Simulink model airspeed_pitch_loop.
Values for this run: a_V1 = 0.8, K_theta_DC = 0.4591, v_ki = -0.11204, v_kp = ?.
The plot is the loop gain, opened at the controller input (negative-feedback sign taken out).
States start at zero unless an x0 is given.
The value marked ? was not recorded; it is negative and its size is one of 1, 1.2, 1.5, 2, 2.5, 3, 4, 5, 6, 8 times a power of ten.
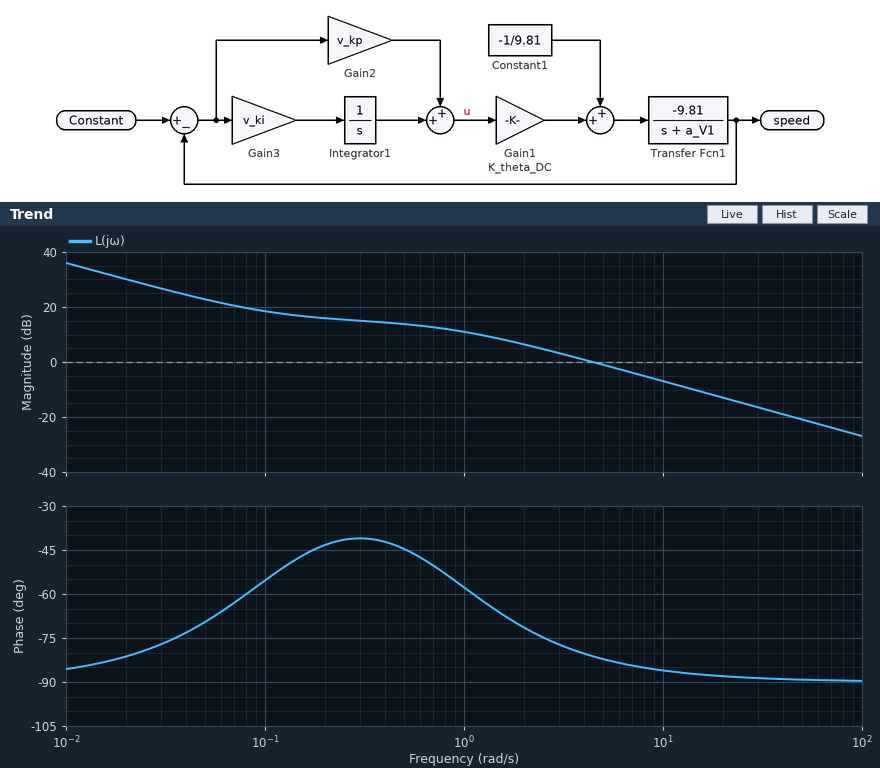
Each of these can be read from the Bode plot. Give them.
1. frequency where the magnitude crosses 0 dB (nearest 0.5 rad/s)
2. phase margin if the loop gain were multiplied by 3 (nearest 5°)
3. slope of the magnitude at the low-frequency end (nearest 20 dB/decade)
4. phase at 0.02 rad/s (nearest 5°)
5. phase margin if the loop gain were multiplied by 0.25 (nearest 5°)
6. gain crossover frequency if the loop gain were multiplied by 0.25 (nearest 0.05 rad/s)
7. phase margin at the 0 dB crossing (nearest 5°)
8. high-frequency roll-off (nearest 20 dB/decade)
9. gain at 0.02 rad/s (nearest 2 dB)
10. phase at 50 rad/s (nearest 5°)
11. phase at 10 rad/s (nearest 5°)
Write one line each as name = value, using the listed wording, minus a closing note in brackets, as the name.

frequency where the magnitude crosses 0 dB = 4.5 rad/s
phase margin if the loop gain were multiplied by 3 = 95°
slope of the magnitude at the low-frequency end = -20 dB/decade
phase at 0.02 rad/s = -80°
phase margin if the loop gain were multiplied by 0.25 = 125°
gain crossover frequency if the loop gain were multiplied by 0.25 = 0.80 rad/s
phase margin at the 0 dB crossing = 100°
high-frequency roll-off = -20 dB/decade
gain at 0.02 rad/s = 30 dB
phase at 50 rad/s = -90°
phase at 10 rad/s = -85°
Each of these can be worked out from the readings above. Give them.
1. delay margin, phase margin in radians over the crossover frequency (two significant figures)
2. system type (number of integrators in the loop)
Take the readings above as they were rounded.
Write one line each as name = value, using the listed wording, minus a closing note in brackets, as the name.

delay margin, phase margin in radians over the crossover frequency = 0.39 s
system type = 1
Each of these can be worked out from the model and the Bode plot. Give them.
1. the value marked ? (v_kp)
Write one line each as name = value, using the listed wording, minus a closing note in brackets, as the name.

the value marked ? = -1
